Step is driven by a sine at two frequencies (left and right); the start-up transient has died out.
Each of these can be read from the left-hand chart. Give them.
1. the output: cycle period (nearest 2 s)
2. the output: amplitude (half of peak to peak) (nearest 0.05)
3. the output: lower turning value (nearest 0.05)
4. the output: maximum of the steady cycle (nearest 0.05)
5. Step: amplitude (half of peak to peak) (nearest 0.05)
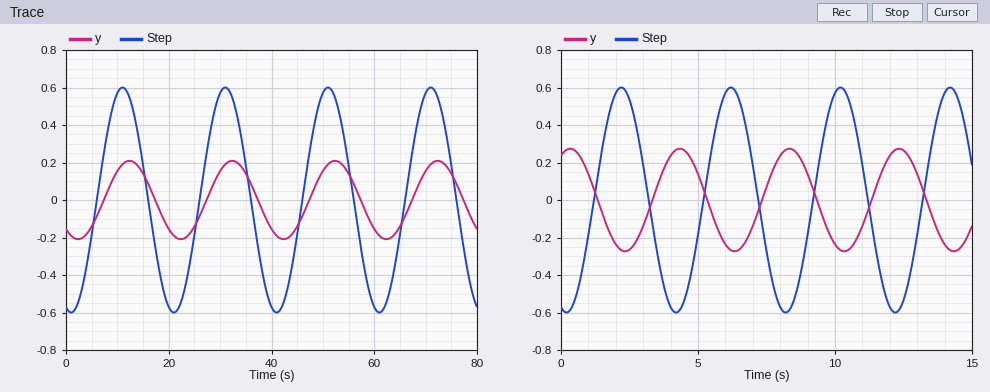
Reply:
20 s
0.20
-0.20
0.20
0.60
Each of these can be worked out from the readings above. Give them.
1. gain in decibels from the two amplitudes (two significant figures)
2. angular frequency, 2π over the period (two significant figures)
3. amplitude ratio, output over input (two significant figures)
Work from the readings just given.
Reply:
-9.5 dB
0.31 rad/s
0.33
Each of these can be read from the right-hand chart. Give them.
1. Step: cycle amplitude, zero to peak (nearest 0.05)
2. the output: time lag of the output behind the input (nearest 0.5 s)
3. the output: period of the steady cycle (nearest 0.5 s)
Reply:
0.60
2.0 s
4.0 s
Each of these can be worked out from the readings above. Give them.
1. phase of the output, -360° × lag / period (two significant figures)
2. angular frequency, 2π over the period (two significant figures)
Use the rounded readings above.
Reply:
-180°
1.6 rad/s
